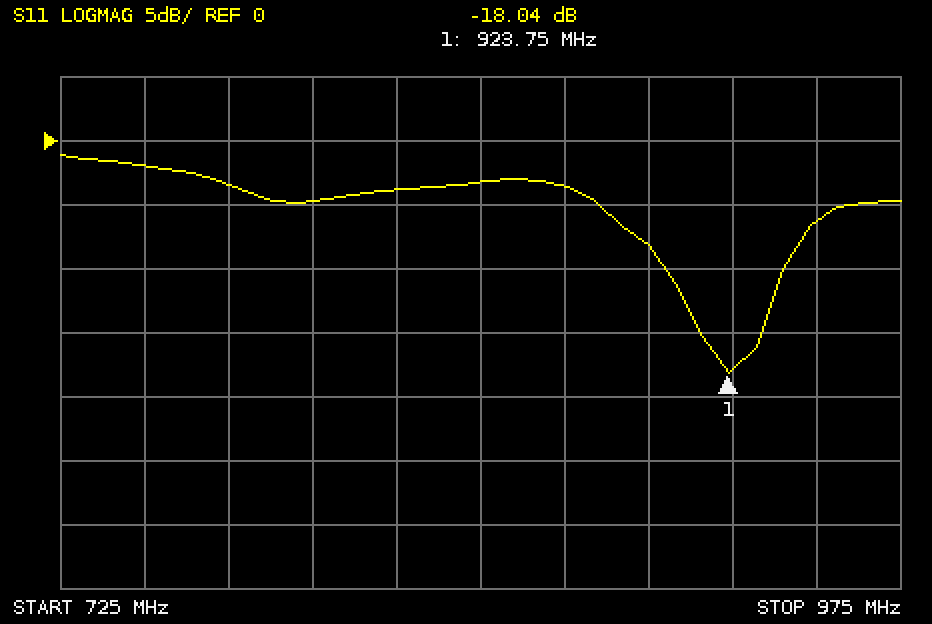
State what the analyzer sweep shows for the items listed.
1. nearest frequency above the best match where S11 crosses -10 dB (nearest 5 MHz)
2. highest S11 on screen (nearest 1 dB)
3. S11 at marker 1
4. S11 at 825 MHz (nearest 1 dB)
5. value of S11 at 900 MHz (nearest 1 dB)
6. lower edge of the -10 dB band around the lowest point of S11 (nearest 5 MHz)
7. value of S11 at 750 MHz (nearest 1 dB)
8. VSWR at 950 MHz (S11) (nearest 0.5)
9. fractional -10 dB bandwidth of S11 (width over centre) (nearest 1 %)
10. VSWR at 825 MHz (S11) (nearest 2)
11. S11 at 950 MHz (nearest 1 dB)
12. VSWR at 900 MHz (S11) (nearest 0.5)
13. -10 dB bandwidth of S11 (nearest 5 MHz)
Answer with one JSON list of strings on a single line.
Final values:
["940 MHz", "-1 dB", "-18.04 dB", "-4 dB", "-8 dB", "905 MHz", "-2 dB", "3.0", "4 %", "4", "-6 dB", "2.5", "35 MHz"]
